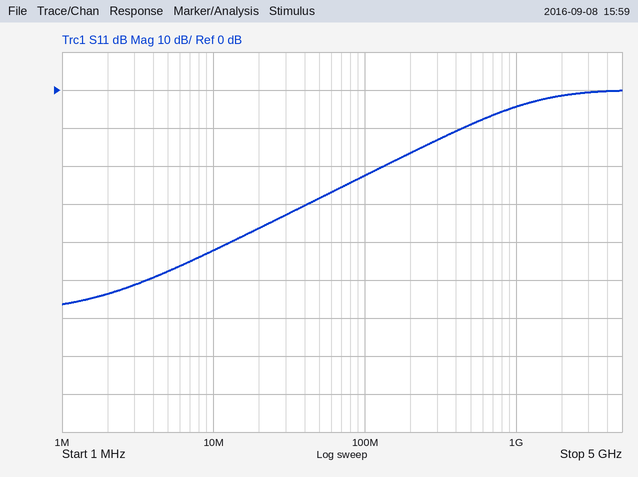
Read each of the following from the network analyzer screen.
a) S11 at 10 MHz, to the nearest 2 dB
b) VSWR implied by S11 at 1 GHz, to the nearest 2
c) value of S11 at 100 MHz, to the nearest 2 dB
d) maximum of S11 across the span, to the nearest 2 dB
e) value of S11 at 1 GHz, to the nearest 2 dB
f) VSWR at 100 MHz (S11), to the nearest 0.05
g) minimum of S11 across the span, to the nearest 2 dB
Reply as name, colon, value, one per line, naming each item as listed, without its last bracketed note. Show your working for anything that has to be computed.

S11 at 10 MHz, to the nearest 2 dB: -42 dB
VSWR implied by S11 at 1 GHz, to the nearest 2: |Γ| = 10^(-4/20) = 0.6310; VSWR = (1 + 0.6310)/(1 − 0.6310) ≈ 4
value of S11 at 100 MHz, to the nearest 2 dB: -22 dB
maximum of S11 across the span, to the nearest 2 dB: 0 dB
value of S11 at 1 GHz, to the nearest 2 dB: -4 dB
VSWR at 100 MHz (S11), to the nearest 0.05: |Γ| = 10^(-22/20) = 0.0794; VSWR = (1 + 0.0794)/(1 − 0.0794) ≈ 1.17, so 1.15 to the nearest 0.05
minimum of S11 across the span, to the nearest 2 dB: -56 dB
